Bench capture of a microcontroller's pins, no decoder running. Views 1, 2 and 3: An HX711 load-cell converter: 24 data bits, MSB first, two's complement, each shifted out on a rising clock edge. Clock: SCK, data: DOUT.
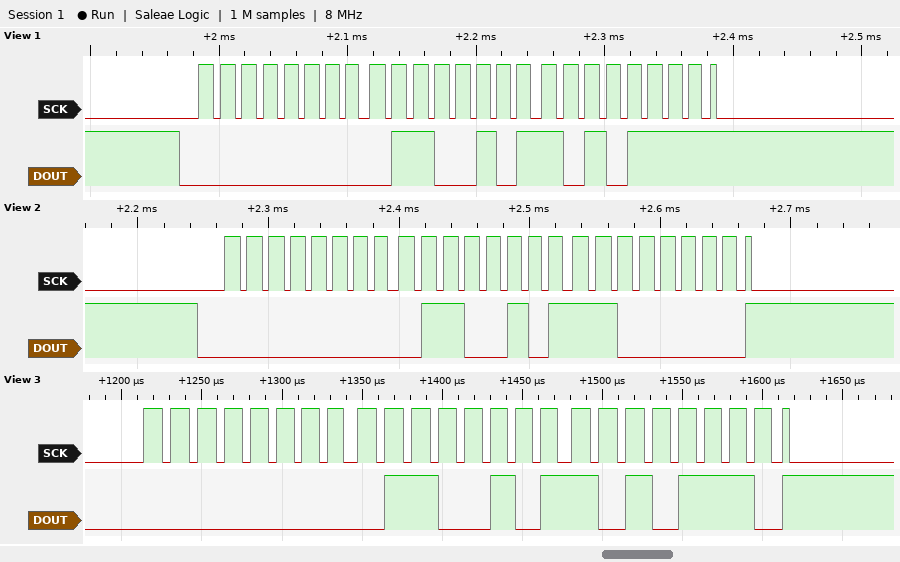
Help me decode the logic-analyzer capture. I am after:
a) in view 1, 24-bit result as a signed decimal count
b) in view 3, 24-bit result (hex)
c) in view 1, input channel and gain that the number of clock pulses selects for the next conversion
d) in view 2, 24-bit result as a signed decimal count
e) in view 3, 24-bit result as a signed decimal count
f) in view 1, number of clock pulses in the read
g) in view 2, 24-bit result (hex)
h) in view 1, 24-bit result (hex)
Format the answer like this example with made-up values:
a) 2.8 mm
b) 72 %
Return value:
a) 26031
b) 0x0065AE
c) channel A, gain 128
d) 26048
e) 26030
f) 25
g) 0x0065C0
h) 0x0065AF
